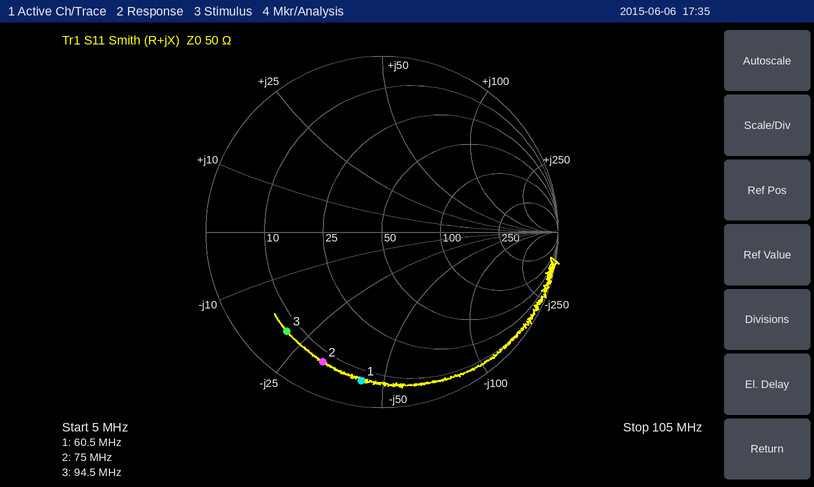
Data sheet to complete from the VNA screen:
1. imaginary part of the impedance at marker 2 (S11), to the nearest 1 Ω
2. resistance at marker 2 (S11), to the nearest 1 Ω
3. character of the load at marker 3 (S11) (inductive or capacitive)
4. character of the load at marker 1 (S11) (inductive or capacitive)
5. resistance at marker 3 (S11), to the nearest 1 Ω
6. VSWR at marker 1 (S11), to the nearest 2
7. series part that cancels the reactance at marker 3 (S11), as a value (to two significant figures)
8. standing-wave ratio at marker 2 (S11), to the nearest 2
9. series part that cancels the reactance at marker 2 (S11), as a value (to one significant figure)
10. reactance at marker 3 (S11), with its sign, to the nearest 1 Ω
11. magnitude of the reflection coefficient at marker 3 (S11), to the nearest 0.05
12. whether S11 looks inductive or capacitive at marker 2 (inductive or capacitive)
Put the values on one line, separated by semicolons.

-32 Ω; 7 Ω; capacitive; capacitive; 7 Ω; 12; 35 nH; 10; 70 nH; -21 Ω; 0.80; capacitive
